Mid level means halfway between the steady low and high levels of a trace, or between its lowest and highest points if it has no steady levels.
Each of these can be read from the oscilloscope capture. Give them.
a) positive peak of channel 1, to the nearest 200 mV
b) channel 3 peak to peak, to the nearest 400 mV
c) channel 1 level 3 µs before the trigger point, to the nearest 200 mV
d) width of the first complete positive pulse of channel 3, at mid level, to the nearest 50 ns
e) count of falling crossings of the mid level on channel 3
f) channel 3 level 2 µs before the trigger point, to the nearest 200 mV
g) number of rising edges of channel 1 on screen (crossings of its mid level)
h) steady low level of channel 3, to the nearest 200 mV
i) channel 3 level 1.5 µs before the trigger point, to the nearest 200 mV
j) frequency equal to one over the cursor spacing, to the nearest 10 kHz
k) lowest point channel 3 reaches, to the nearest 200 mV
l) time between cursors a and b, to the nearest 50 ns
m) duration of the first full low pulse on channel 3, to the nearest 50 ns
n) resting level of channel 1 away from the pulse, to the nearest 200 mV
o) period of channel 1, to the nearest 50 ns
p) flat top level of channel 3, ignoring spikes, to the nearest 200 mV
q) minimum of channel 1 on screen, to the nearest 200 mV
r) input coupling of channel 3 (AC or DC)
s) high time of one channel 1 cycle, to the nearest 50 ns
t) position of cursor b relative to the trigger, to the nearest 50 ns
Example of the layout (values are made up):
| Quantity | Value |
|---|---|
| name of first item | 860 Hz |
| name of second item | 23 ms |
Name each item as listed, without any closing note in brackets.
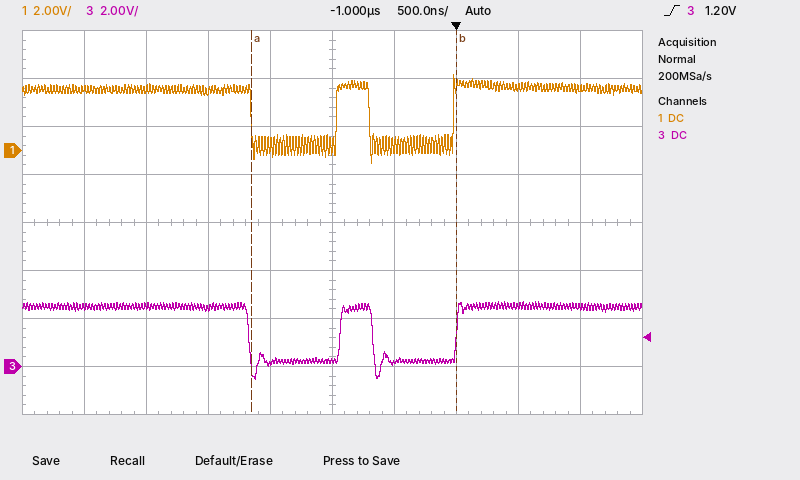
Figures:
| Quantity | Value |
|---|---|
| positive peak of channel 1, to the nearest 200 mV | 3.2 V |
| channel 3 peak to peak, to the nearest 400 mV | 3.2 V |
| channel 1 level 3 µs before the trigger point, to the nearest 200 mV | 2.6 V |
| width of the first complete positive pulse of channel 3, at mid level, to the nearest 50 ns | 250 ns |
| count of falling crossings of the mid level on channel 3 | 2 |
| channel 3 level 2 µs before the trigger point, to the nearest 200 mV | 2.4 V |
| number of rising edges of channel 1 on screen | 2 |
| steady low level of channel 3, to the nearest 200 mV | 200 mV |
| channel 3 level 1.5 µs before the trigger point, to the nearest 200 mV | 200 mV |
| frequency equal to one over the cursor spacing, to the nearest 10 kHz | 610 kHz |
| lowest point channel 3 reaches, to the nearest 200 mV | -600 mV |
| time between cursors a and b, to the nearest 50 ns | 1.65 µs |
| duration of the first full low pulse on channel 3, to the nearest 50 ns | 750 ns |
| resting level of channel 1 away from the pulse, to the nearest 200 mV | 2.6 V |
| period of channel 1, to the nearest 50 ns | 950 ns |
| flat top level of channel 3, ignoring spikes, to the nearest 200 mV | 2.4 V |
| minimum of channel 1 on screen, to the nearest 200 mV | -600 mV |
| input coupling of channel 3 | DC |
| high time of one channel 1 cycle, to the nearest 50 ns | 250 ns |
| position of cursor b relative to the trigger, to the nearest 50 ns | 0 ns |
